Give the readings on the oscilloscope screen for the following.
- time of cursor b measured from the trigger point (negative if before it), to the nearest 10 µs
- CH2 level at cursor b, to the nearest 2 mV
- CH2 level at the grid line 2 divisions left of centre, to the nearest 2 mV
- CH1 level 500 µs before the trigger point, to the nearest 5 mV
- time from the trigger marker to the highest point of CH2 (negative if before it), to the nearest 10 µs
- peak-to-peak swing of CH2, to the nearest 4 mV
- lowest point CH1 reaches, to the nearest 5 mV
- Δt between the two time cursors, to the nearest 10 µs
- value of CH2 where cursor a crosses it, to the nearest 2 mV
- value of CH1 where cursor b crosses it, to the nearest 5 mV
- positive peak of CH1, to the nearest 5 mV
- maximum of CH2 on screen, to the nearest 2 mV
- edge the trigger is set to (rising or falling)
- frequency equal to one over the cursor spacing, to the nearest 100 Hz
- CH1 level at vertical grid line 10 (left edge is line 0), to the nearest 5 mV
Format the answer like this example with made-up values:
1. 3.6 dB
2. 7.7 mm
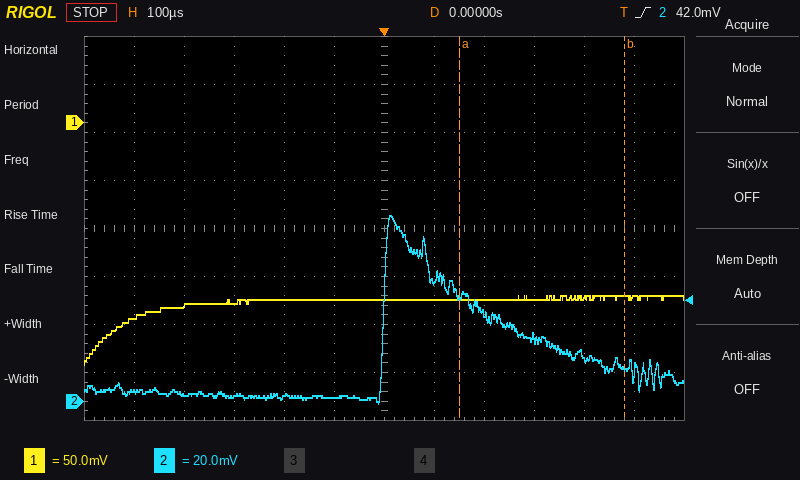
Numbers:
1. +480 µs
2. 14 mV
3. 2 mV
4. -200 mV
5. +10 µs
6. 80 mV
7. -250 mV
8. 330 µs
9. 44 mV
10. -180 mV
11. -180 mV
12. 78 mV
13. rising
14. 3.0 kHz
15. -180 mV
